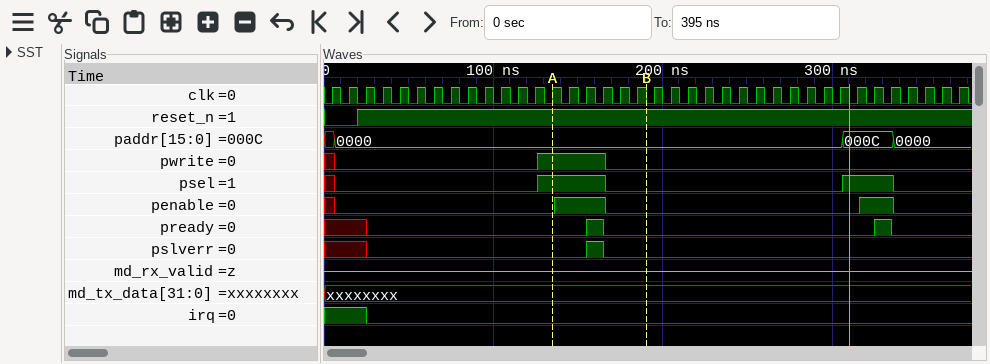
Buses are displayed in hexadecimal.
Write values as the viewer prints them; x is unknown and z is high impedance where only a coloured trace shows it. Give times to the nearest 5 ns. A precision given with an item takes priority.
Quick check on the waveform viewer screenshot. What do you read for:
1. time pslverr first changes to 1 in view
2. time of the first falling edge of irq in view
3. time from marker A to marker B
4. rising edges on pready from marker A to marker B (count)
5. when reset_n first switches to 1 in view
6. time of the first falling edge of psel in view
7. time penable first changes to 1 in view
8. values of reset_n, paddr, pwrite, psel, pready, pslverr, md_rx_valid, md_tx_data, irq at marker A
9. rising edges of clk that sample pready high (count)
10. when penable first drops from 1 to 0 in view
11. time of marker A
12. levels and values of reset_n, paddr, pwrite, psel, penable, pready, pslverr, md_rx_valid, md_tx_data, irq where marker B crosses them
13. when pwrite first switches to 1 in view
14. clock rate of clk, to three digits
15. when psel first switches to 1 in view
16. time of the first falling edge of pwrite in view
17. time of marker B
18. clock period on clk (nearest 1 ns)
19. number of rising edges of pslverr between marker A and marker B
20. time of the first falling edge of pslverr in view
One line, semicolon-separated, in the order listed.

155 ns; 25 ns; 55 ns; 1; 20 ns; 165 ns; 135 ns; reset_n=1, paddr=0000, pwrite=1, psel=1, pready=0, pslverr=0, md_rx_valid=z, md_tx_data=xxxxxxxx, irq=0; 2; 165 ns; 135 ns; reset_n=1, paddr=0000, pwrite=0, psel=0, penable=0, pready=0, pslverr=0, md_rx_valid=z, md_tx_data=xxxxxxxx, irq=0; 125 ns; 100 MHz; 125 ns; 165 ns; 190 ns; 10 ns; 1; 165 ns
